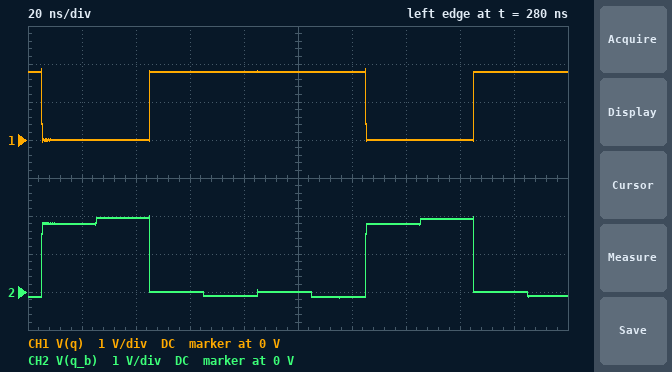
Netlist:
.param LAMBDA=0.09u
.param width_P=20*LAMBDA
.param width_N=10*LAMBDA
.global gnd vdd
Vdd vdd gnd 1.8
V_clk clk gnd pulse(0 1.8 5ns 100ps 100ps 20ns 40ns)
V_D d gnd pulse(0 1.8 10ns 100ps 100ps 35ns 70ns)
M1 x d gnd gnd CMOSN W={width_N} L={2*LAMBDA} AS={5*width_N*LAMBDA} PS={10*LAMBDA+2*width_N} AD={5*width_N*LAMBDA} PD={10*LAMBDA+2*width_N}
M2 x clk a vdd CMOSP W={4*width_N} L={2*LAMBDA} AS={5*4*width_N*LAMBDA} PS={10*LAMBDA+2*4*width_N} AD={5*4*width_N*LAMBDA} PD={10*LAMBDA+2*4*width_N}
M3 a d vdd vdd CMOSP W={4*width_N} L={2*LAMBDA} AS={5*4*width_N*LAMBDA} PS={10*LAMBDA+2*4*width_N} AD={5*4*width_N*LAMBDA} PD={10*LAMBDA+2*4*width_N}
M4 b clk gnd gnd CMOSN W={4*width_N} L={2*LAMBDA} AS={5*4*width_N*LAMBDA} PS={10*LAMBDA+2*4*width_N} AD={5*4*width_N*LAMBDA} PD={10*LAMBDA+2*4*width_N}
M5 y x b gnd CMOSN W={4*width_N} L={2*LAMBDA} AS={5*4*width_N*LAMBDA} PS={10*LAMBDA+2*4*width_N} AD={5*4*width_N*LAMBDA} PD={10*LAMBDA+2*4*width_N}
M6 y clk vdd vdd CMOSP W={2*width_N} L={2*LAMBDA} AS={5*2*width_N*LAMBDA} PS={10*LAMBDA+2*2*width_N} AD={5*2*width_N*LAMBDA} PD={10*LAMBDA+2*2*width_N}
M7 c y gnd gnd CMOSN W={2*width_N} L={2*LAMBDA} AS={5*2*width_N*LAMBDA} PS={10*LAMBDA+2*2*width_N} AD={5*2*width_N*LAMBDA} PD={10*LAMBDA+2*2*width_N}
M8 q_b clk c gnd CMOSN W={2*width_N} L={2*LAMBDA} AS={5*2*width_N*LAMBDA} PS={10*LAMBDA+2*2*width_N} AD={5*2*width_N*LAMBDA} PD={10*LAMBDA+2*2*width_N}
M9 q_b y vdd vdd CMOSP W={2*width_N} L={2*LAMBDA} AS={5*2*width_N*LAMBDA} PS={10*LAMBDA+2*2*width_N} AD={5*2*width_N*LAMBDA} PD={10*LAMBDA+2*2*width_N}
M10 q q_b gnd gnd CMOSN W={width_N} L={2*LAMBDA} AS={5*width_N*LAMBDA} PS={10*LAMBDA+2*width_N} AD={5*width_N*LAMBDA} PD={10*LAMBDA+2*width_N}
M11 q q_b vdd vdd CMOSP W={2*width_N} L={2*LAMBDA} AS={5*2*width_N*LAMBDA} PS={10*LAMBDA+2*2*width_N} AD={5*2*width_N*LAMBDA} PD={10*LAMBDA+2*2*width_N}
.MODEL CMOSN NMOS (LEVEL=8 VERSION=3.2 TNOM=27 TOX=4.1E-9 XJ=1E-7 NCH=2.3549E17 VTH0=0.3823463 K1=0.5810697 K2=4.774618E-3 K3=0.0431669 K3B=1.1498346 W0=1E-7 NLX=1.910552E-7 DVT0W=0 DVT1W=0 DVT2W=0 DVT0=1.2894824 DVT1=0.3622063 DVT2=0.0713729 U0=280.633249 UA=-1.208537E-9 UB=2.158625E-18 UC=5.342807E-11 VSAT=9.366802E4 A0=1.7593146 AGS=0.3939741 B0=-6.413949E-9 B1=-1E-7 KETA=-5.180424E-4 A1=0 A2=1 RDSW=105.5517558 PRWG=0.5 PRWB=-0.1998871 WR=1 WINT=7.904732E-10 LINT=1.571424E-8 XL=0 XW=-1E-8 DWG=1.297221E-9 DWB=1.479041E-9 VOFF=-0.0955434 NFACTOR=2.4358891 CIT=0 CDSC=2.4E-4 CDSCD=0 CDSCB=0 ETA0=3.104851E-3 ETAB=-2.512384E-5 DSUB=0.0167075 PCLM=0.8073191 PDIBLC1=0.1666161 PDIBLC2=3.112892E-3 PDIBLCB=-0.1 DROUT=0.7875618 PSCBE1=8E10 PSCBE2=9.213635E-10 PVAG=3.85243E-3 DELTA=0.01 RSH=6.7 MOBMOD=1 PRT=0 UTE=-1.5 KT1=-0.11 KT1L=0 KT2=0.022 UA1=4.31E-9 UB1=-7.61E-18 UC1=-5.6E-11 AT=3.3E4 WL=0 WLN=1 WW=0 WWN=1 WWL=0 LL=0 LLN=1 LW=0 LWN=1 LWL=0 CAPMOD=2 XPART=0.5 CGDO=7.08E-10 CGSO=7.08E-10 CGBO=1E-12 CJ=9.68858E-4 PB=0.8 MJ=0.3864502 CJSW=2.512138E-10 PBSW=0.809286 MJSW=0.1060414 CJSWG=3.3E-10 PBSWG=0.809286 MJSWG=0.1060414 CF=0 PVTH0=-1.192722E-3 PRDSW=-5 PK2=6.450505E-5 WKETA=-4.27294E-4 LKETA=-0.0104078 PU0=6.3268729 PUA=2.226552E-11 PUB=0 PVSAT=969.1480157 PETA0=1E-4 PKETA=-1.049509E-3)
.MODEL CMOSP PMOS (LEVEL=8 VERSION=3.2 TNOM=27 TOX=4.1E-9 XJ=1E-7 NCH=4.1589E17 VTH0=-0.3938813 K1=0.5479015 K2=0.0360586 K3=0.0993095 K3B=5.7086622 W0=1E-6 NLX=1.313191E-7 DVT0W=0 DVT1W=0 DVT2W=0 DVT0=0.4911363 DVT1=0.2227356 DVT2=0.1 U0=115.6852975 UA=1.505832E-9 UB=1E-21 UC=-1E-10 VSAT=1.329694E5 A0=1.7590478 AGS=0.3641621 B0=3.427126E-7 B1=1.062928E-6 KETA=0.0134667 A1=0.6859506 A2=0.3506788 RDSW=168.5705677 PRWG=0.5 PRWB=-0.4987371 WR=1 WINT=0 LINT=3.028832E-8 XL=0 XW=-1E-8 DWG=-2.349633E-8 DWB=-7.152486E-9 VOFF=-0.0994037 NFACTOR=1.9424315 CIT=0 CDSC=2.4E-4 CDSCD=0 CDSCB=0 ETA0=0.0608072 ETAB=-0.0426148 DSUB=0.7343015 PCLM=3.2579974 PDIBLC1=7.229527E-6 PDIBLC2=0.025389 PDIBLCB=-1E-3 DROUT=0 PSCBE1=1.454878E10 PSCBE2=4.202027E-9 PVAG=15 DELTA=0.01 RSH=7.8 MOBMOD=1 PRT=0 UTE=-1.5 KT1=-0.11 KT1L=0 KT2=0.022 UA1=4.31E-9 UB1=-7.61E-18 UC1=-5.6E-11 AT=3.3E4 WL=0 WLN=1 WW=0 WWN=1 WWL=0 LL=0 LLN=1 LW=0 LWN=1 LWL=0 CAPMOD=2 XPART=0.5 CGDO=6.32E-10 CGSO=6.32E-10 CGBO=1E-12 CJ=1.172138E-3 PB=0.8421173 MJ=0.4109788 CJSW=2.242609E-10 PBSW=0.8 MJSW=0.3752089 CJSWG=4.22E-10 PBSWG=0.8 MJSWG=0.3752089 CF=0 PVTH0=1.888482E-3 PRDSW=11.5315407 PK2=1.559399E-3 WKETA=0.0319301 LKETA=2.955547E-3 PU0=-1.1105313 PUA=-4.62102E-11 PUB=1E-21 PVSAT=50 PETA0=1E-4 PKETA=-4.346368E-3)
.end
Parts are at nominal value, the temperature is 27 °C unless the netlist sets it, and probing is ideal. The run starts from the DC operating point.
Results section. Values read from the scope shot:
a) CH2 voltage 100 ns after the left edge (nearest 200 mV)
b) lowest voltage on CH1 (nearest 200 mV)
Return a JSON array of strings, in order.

["0 V", "0 V"]
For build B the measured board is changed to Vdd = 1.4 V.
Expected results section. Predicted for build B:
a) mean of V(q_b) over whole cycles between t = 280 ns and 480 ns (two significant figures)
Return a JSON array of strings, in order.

["440 mV"]
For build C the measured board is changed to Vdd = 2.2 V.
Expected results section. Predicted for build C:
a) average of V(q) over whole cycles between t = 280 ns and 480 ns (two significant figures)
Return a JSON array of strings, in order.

["1.5 V"]
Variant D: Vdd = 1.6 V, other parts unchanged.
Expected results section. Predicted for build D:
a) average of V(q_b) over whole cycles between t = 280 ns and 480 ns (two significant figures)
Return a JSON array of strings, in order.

["510 mV"]
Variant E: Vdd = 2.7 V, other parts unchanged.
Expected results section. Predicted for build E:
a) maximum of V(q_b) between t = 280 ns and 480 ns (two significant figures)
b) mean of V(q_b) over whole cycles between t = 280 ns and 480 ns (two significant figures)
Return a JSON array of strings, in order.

["2.9 V", "1.4 V"]
